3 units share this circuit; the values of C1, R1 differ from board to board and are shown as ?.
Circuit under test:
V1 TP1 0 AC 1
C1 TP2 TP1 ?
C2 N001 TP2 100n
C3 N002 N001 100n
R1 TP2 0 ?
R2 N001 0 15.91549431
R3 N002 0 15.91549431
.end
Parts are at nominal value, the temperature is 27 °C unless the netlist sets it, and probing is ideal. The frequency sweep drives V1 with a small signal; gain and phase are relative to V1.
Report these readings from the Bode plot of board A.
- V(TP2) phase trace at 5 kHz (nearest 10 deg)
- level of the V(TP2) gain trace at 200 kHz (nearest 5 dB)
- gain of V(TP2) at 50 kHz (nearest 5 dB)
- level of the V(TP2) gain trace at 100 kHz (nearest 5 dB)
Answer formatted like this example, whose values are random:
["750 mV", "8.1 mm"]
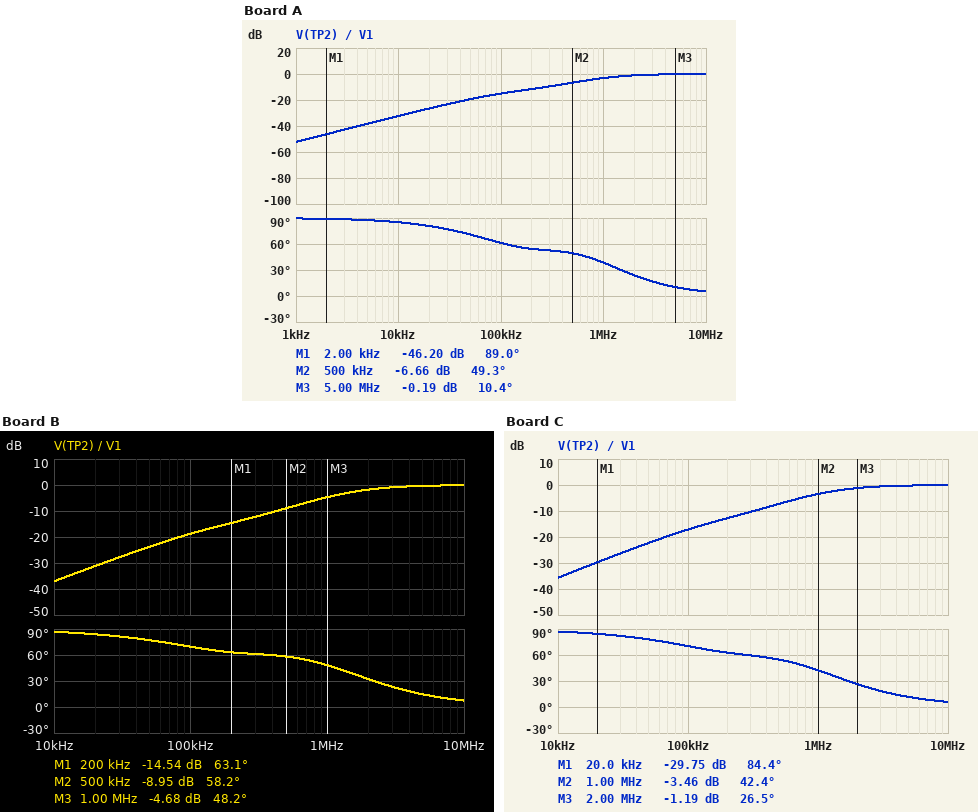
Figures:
["90 deg", "-10 dB", "-20 dB", "-15 dB"]
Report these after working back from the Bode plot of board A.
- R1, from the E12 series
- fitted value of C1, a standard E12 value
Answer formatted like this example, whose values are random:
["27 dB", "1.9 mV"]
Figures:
["10 Ω", "39 nF"]
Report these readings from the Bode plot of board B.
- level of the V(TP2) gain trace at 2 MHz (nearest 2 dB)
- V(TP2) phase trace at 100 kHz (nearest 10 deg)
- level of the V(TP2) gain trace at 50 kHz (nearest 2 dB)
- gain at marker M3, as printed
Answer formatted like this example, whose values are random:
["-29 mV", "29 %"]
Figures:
["-2 dB", "70 deg", "-24 dB", "-4.68 dB"]
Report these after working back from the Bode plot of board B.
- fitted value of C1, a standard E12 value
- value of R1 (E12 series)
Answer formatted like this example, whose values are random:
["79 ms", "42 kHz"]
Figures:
["33 nF", "6.8 Ω"]
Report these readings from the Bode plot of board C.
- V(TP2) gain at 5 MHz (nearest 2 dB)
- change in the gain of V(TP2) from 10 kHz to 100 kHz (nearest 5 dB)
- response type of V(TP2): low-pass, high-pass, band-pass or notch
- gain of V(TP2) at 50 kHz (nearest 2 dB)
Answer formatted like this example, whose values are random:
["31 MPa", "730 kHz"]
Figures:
["0 dB", "20 dB", "high-pass", "-22 dB"]
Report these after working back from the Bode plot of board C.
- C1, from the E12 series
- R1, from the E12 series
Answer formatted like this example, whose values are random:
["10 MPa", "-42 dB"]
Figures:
["47 nF", "5.6 Ω"]
